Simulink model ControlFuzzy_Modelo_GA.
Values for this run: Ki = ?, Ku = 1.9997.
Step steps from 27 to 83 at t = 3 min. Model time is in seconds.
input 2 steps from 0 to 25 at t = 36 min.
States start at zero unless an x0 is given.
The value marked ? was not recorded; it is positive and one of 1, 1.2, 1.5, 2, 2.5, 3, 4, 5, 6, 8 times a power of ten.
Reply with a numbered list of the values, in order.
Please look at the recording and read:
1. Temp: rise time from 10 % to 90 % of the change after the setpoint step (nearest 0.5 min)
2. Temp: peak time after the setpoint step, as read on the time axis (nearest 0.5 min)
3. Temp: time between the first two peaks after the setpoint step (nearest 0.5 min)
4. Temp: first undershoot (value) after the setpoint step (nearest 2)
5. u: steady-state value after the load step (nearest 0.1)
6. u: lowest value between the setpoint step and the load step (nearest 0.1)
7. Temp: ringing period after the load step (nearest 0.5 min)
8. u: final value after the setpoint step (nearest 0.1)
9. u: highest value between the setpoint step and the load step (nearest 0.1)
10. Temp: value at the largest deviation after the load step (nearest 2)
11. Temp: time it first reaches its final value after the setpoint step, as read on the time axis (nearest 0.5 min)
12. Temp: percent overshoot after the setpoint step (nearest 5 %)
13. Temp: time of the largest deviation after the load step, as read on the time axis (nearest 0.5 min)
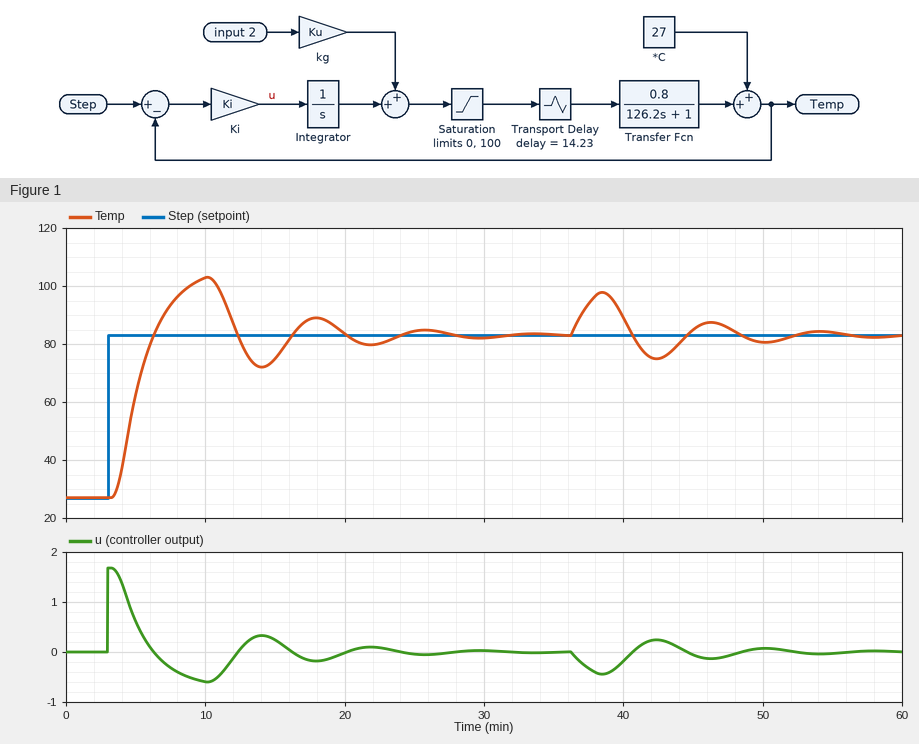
1. 2.0 min
2. 10.0 min
3. 8.0 min
4. 72
5. 0.0
6. -0.6
7. 8.0 min
8. 0.0
9. 1.7
10. 98
11. 6.5 min
12. 35 %
13. 38.5 min
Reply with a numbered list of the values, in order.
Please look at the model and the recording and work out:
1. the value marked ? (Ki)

1. 0.03
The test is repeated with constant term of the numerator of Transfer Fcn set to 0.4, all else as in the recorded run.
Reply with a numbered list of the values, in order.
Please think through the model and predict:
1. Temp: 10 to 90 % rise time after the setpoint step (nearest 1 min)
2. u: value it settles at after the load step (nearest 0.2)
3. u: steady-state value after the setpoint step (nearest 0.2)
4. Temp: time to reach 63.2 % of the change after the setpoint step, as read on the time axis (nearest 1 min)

1. 5 min
2. 0.4
3. 0.4
4. 6 min
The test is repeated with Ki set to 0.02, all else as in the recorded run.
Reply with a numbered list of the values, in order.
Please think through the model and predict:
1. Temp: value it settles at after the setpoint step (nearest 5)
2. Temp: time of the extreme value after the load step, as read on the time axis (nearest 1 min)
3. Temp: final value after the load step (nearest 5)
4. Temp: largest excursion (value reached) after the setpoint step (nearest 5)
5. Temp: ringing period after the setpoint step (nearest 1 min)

1. 85
2. 39 min
3. 85
4. 100
5. 10 min
